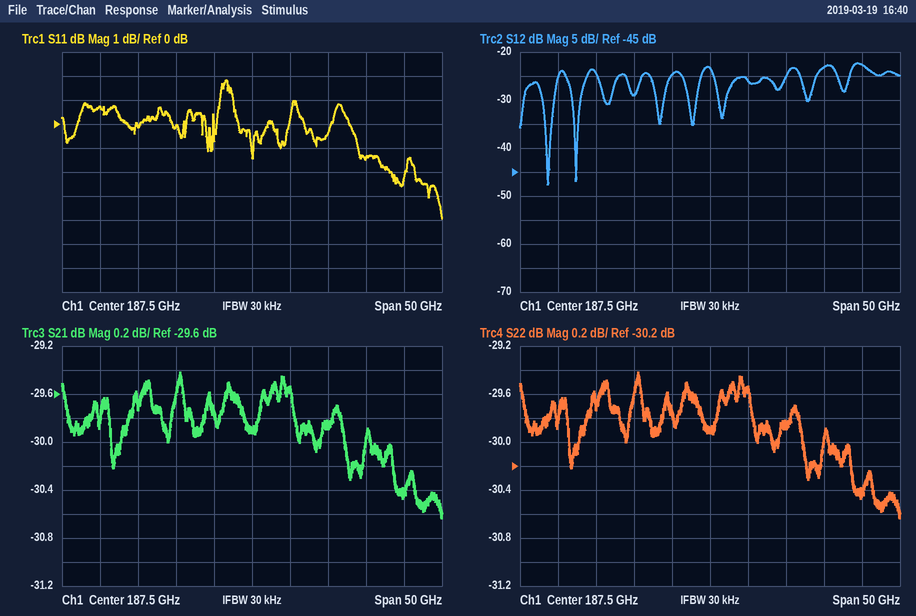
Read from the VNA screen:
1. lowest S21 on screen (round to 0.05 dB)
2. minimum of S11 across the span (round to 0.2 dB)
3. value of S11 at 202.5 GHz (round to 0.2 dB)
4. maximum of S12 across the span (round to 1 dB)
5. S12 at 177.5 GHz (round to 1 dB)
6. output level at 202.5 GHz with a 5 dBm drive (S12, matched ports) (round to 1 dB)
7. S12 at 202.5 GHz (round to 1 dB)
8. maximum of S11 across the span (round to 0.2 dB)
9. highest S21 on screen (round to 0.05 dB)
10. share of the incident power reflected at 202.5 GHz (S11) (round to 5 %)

-30.65 dB
-4.0 dB
-1.4 dB
-22 dB
-29 dB
-18 dBm
-23 dB
1.8 dB
-29.40 dB
70 %
